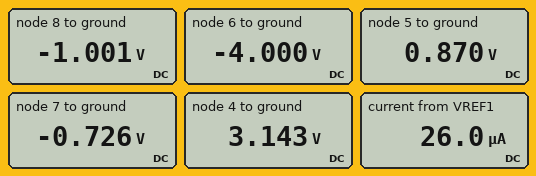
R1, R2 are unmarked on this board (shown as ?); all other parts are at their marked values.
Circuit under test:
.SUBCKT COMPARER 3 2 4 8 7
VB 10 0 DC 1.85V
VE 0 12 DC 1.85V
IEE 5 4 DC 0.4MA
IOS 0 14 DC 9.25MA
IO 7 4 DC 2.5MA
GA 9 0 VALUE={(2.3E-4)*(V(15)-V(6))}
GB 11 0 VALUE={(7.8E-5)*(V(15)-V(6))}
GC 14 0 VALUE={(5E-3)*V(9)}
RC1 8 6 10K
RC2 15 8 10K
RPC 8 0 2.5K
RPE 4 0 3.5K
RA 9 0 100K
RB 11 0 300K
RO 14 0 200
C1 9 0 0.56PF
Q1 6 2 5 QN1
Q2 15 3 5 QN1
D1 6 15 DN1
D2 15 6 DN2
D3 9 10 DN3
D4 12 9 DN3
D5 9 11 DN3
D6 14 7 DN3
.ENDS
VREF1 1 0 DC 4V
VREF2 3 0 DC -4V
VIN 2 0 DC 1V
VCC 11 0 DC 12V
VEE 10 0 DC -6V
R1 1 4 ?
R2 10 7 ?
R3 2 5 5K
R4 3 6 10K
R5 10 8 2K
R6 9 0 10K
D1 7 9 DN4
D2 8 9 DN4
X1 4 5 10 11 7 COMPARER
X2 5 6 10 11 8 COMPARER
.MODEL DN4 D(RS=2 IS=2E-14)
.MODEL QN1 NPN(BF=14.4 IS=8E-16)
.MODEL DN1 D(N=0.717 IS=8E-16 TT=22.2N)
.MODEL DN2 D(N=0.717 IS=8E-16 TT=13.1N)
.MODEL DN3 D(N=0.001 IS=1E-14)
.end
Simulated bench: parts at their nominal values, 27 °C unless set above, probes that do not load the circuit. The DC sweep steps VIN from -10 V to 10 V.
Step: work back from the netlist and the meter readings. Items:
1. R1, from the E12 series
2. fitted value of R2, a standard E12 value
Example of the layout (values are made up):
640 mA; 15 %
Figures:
33 kΩ; 4.7 kΩ
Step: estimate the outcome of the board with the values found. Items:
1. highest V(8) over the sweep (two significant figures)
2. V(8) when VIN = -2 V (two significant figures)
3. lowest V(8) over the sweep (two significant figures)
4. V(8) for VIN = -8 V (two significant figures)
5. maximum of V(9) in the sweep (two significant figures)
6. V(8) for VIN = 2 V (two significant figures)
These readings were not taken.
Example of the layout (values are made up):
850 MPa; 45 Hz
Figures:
2.3 V; -1.0 V; -1.0 V; 2.3 V; 2.2 V; -1.0 V
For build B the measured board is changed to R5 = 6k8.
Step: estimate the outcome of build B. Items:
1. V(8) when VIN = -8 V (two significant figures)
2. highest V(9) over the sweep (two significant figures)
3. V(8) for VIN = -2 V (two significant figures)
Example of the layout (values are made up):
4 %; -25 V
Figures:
2.9 V; 2.3 V; -660 mV
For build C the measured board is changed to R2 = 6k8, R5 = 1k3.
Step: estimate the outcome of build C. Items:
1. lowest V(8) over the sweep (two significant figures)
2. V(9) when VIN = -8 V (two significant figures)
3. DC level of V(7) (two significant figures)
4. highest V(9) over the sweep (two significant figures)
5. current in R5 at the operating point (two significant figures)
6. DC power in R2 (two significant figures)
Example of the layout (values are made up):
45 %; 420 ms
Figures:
-1.2 V; 1.4 V; -660 mV; 2.3 V; 3.7 mA; 4.2 mW
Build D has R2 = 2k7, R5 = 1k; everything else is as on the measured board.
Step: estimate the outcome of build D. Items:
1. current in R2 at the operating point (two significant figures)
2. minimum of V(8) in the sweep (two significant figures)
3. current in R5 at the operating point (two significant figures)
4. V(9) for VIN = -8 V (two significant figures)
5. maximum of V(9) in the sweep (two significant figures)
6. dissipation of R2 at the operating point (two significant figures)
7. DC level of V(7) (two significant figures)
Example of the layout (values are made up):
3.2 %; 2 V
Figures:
1.9 mA; -1.4 V; 4.6 mA; 1.1 V; 1.9 V; 9.7 mW; -880 mV
